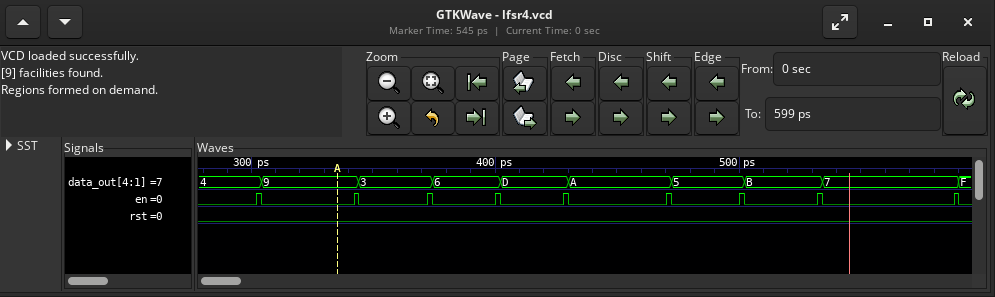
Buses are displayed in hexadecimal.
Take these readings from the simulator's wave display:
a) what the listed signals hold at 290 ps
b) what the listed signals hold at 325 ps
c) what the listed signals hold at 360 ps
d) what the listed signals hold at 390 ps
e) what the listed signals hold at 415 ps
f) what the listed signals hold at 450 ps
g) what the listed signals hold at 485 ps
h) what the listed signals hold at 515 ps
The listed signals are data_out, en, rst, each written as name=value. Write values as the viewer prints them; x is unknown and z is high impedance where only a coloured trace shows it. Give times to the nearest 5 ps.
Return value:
data_out=4, en=0, rst=0
data_out=9, en=0, rst=0
data_out=3, en=0, rst=0
data_out=6, en=0, rst=0
data_out=D, en=0, rst=0
data_out=A, en=0, rst=0
data_out=5, en=0, rst=0
data_out=B, en=0, rst=0
